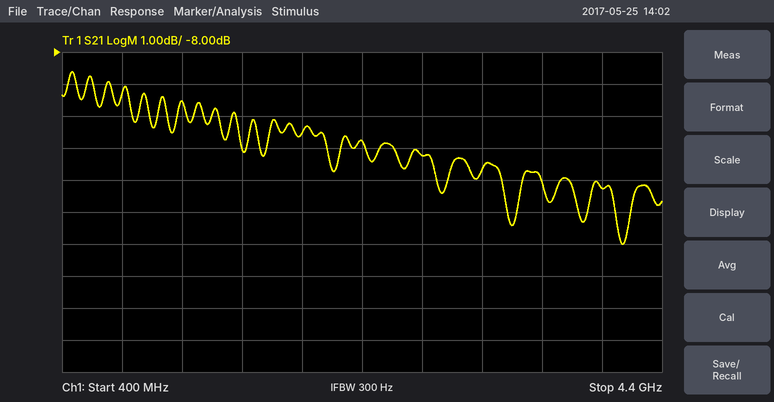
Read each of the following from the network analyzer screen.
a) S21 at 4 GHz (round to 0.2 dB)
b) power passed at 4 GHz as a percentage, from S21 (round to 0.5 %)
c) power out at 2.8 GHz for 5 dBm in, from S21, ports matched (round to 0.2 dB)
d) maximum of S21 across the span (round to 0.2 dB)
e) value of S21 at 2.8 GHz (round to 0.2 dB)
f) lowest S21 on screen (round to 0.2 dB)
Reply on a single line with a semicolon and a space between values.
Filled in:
-12.2 dB; 6.0 %; -6.2 dBm; -8.6 dB; -11.2 dB; -14.0 dB
